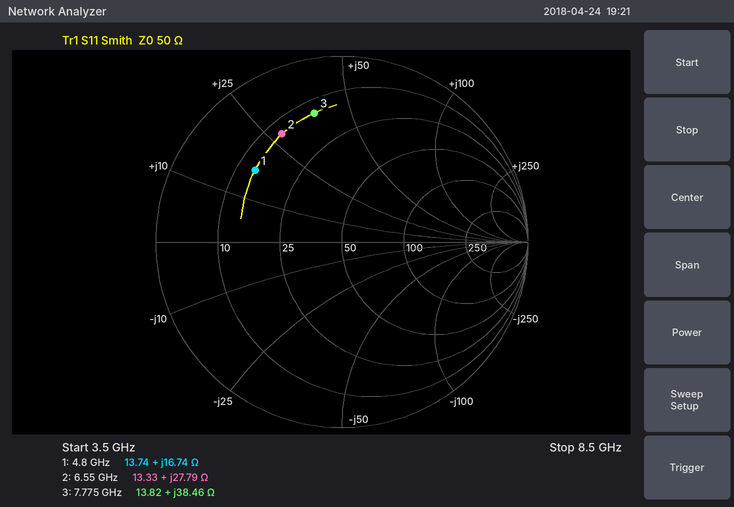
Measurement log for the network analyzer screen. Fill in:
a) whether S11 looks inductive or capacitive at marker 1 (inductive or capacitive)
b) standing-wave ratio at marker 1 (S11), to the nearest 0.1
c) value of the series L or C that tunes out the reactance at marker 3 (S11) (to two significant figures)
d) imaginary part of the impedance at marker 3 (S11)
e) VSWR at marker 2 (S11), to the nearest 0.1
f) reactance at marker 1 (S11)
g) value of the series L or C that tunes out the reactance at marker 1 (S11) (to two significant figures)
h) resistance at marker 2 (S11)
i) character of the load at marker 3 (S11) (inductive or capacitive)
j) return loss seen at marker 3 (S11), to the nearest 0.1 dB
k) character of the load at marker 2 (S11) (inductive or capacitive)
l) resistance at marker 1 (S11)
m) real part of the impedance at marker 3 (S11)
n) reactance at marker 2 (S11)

inductive
4.1
530 fF
+38.46 Ω
5.0
+16.74 Ω
2.0 pF
13.33 Ω
inductive
3.0 dB
inductive
13.74 Ω
13.82 Ω
+27.79 Ω
